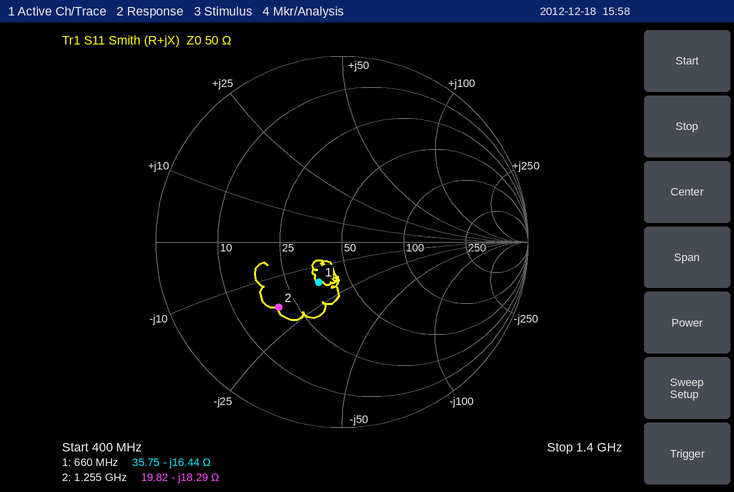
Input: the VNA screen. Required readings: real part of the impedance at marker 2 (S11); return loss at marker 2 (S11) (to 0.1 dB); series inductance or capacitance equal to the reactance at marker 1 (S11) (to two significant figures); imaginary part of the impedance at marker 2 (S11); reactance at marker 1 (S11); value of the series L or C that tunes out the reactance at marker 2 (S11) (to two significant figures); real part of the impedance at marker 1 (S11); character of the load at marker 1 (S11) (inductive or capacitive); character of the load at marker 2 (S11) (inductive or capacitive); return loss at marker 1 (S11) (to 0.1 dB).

19.82 Ω
6.2 dB
15 pF
-18.29 Ω
-16.44 Ω
2.3 nH
35.75 Ω
capacitive
capacitive
12.1 dB
